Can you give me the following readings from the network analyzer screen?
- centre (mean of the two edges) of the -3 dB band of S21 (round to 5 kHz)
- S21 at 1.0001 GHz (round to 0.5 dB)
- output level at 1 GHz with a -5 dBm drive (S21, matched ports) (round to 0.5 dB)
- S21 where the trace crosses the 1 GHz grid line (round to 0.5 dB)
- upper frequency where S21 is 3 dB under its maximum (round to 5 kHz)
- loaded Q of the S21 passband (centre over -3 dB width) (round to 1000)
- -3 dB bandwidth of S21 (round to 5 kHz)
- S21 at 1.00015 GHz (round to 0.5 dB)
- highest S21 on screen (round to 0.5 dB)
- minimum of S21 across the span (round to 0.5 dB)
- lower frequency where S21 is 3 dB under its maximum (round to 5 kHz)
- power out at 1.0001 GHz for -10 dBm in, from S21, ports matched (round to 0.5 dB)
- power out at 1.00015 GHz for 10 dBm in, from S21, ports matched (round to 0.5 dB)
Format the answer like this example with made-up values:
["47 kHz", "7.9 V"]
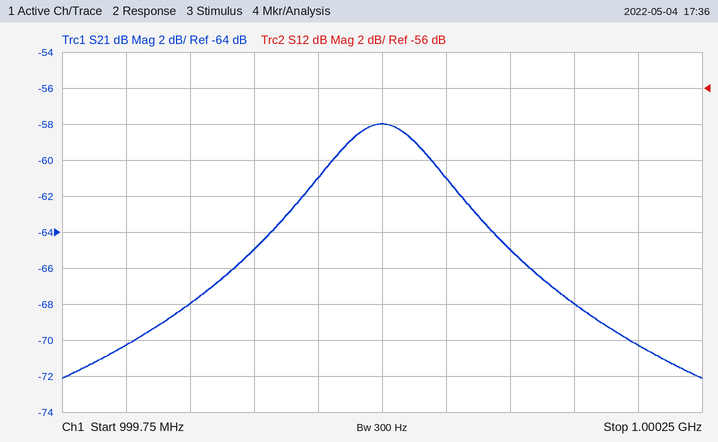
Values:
["1.000000 GHz", "-65.0 dB", "-63.0 dBm", "-58.0 dB", "1.000050 GHz", "10000", "100 kHz", "-68.0 dB", "-58.0 dB", "-72.0 dB", "999.950 MHz", "-75.0 dBm", "-58.0 dBm"]
